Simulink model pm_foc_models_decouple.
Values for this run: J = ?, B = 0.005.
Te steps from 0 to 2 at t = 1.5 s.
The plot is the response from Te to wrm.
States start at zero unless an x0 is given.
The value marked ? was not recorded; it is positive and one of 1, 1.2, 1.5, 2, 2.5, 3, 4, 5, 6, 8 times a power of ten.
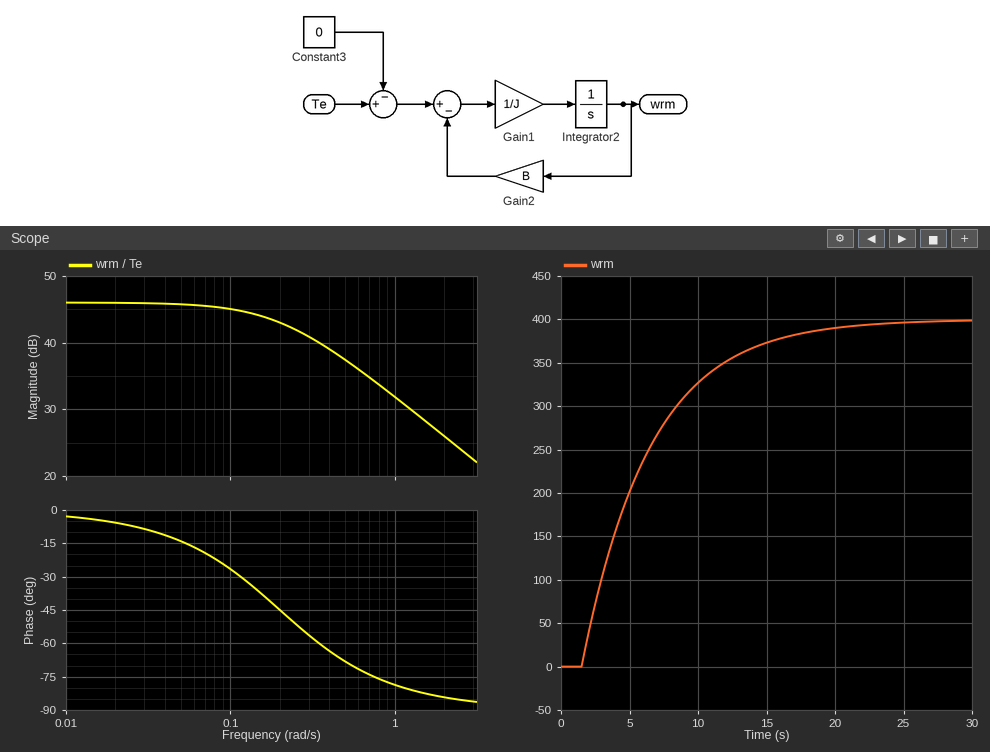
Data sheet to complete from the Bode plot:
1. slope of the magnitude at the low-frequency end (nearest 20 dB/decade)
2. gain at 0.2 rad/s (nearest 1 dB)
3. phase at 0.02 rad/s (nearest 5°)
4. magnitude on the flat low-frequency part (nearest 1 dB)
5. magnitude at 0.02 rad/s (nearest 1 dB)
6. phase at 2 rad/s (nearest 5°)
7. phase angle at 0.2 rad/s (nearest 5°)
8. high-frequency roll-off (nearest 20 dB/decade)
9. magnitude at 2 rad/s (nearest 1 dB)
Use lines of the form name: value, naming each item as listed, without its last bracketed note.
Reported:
slope of the magnitude at the low-frequency end: 0 dB/decade
gain at 0.2 rad/s: 43 dB
phase at 0.02 rad/s: -5°
magnitude on the flat low-frequency part: 46 dB
magnitude at 0.02 rad/s: 46 dB
phase at 2 rad/s: -85°
phase angle at 0.2 rad/s: -45°
high-frequency roll-off: -20 dB/decade
magnitude at 2 rad/s: 26 dB
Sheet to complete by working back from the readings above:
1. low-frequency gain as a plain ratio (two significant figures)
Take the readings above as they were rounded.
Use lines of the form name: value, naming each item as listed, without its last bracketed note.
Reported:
low-frequency gain as a plain ratio: 200
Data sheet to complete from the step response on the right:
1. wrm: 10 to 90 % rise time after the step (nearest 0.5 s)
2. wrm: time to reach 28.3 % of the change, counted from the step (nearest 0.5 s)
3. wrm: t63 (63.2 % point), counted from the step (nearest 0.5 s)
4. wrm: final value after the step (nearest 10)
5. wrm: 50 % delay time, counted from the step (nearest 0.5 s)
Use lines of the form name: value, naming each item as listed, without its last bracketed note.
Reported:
wrm: 10 to 90 % rise time after the step: 11.0 s
wrm: time to reach 28.3 % of the change, counted from the step: 1.5 s
wrm: t63 (63.2 % point), counted from the step: 5.0 s
wrm: final value after the step: 400
wrm: 50 % delay time, counted from the step: 3.5 s
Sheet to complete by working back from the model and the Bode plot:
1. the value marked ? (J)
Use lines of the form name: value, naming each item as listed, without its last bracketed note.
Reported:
the value marked ?: 0.025
